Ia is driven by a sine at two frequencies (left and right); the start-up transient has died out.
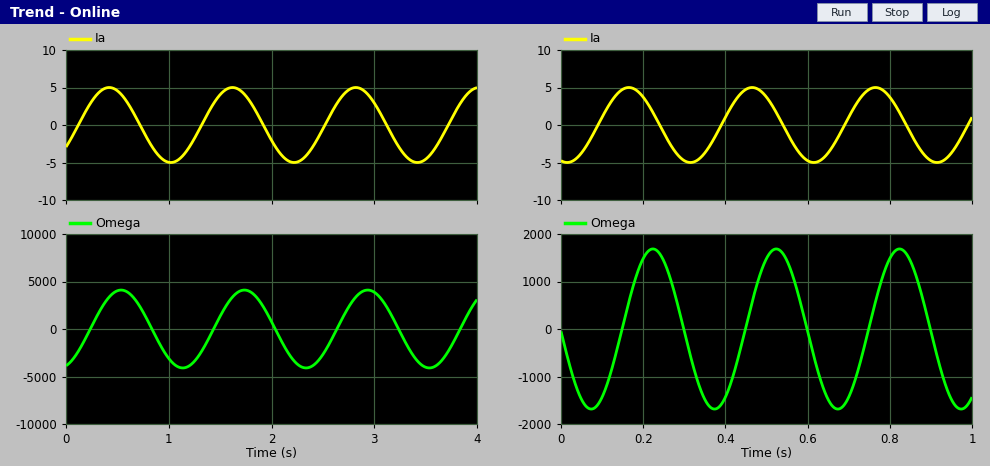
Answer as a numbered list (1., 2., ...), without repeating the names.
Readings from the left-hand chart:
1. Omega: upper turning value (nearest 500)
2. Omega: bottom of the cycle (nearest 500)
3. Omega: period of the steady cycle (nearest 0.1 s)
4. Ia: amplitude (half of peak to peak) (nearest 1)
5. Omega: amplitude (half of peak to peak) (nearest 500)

1. 4000
2. -4000
3. 1.2 s
4. 5
5. 4000
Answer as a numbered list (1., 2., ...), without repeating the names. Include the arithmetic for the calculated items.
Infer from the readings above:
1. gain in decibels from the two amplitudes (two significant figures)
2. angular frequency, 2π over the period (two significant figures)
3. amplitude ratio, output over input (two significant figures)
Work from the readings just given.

1. 20 log10(4000 / 5) = 58 dB
2. 2π / 1.2 = 5.2 rad/s
3. 4000 / 5 = 800
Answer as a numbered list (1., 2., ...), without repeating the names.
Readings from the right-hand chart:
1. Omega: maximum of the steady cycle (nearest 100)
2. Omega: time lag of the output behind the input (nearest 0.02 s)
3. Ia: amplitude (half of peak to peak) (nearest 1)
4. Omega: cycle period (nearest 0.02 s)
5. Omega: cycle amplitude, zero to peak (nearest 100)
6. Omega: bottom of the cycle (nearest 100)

1. 1700
2. 0.06 s
3. 5
4. 0.30 s
5. 1700
6. -1700
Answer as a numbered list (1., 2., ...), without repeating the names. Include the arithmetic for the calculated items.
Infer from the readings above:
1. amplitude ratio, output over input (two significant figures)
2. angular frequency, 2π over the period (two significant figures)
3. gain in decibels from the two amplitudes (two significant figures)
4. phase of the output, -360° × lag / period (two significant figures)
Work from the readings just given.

1. 1700 / 5 = 340
2. 2π / 0.3 = 21 rad/s
3. 20 log10(1700 / 5) = 51 dB
4. -360 × 0.06 / 0.3 = -72°
